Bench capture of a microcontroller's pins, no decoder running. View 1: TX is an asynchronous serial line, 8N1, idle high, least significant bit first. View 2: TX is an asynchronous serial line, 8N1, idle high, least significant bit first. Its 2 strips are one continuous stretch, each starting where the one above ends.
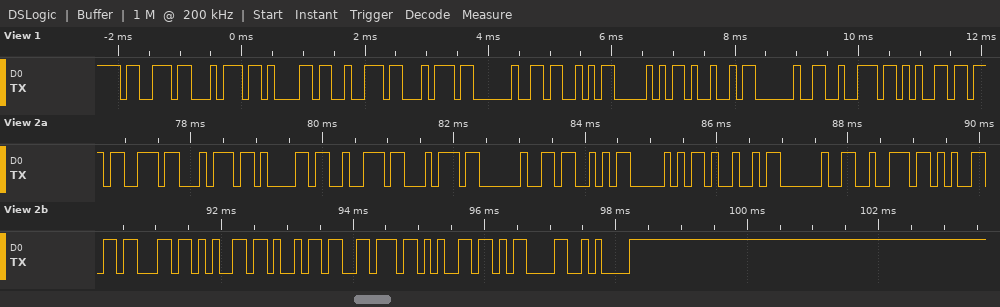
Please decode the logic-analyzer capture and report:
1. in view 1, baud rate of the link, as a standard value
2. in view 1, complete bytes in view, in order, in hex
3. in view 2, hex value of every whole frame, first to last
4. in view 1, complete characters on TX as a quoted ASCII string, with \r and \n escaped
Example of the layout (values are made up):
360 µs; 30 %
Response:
9600 baud; 73 74 61 72 74 20 53 50 49 20 72 65; 73 74 61 72 74 20 53 50 49 20 72 65 63 65 69 76 65 0D 0A; "start SPI re"
